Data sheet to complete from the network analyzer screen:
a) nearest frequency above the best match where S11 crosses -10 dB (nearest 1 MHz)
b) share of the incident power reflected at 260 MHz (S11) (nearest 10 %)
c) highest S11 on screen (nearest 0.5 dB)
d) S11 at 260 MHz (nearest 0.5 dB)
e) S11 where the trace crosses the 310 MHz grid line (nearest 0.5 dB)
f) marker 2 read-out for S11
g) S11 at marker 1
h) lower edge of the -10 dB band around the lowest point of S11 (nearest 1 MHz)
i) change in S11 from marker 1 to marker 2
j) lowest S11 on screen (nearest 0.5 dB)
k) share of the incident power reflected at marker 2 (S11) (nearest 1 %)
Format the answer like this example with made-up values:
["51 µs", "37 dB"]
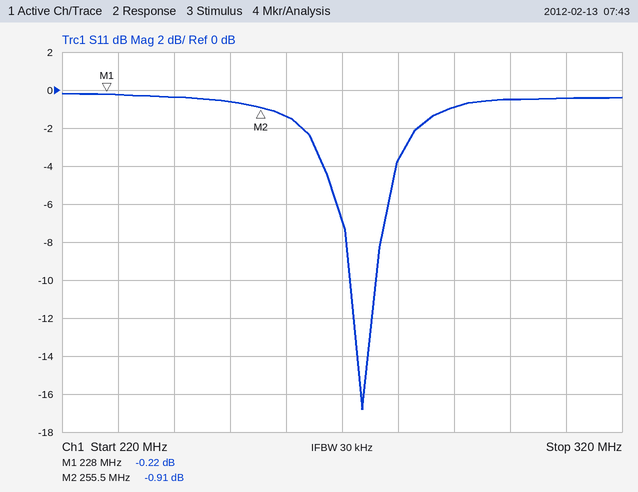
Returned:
["276 MHz", "70 %", "0.0 dB", "-1.5 dB", "-0.5 dB", "-0.91 dB", "-0.22 dB", "271 MHz", "-0.69 dB", "-17.0 dB", "81 %"]
